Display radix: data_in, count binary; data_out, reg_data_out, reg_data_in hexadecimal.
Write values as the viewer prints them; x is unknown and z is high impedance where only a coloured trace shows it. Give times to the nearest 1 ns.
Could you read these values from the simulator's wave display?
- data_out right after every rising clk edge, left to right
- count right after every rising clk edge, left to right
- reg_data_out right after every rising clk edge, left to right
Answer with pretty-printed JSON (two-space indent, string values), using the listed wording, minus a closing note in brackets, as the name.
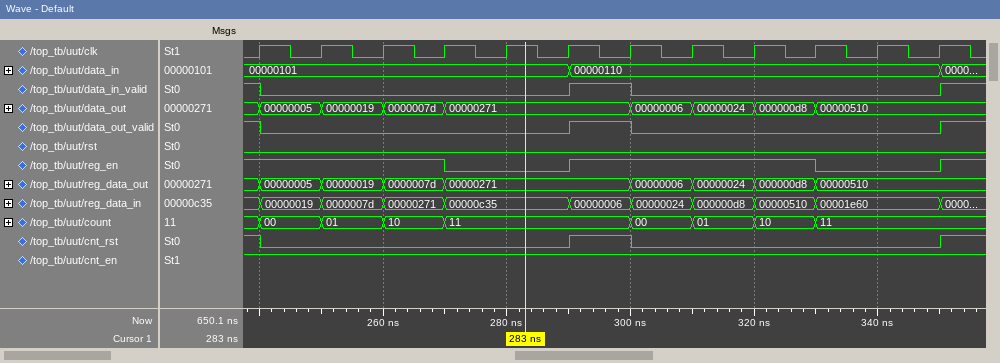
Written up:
{
  "data_out right after every rising clk edge, left to right": "00000005, 00000019, 0000007d, 00000271, 00000271, 00000271, 00000006, 00000024, 000000d8, 00000510, 00000510, 00000510",
  "count right after every rising clk edge, left to right": "00, 01, 10, 11, 11, 11, 00, 01, 10, 11, 11, 11",
  "reg_data_out right after every rising clk edge, left to right": "00000005, 00000019, 0000007d, 00000271, 00000271, 00000271, 00000006, 00000024, 000000d8, 00000510, 00000510, 00000510"
}
